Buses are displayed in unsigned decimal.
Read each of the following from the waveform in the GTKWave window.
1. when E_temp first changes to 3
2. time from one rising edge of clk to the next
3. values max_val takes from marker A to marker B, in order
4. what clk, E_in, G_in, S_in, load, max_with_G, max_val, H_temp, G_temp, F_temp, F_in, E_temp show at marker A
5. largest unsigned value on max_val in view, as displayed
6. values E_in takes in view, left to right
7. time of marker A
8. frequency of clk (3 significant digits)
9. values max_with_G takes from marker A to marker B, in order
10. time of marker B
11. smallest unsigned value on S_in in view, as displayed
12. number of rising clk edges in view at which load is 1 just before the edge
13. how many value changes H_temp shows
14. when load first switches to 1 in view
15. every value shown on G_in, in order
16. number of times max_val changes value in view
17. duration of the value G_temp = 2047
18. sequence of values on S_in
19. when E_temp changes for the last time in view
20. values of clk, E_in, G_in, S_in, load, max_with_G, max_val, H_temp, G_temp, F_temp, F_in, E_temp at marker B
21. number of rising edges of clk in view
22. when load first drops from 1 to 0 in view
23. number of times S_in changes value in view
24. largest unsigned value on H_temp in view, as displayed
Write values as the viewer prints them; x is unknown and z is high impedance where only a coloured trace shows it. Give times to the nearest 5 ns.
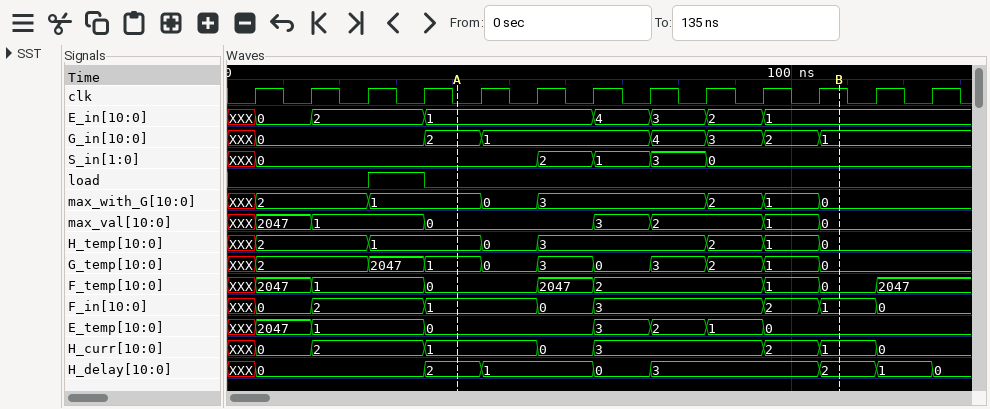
65 ns
10 ns
0, 3, 2, 1, 0
clk=0, E_in=1, G_in=2, S_in=0, load=0, max_with_G=1, max_val=0, H_temp=1, G_temp=1, F_temp=0, F_in=1, E_temp=0
2047
XXX, 0, 2, 1, 4, 3, 2, 1
40 ns
100 MHz
1, 0, 3, 2, 1, 0
110 ns
0
1
7
25 ns
XXX, 0, 2, 1, 4, 3, 2, 1
7
10 ns
XXX, 0, 2, 1, 3, 0
95 ns
clk=1, E_in=1, G_in=1, S_in=0, load=0, max_with_G=0, max_val=0, H_temp=0, G_temp=0, F_temp=0, F_in=1, E_temp=0
13
35 ns
5
3
